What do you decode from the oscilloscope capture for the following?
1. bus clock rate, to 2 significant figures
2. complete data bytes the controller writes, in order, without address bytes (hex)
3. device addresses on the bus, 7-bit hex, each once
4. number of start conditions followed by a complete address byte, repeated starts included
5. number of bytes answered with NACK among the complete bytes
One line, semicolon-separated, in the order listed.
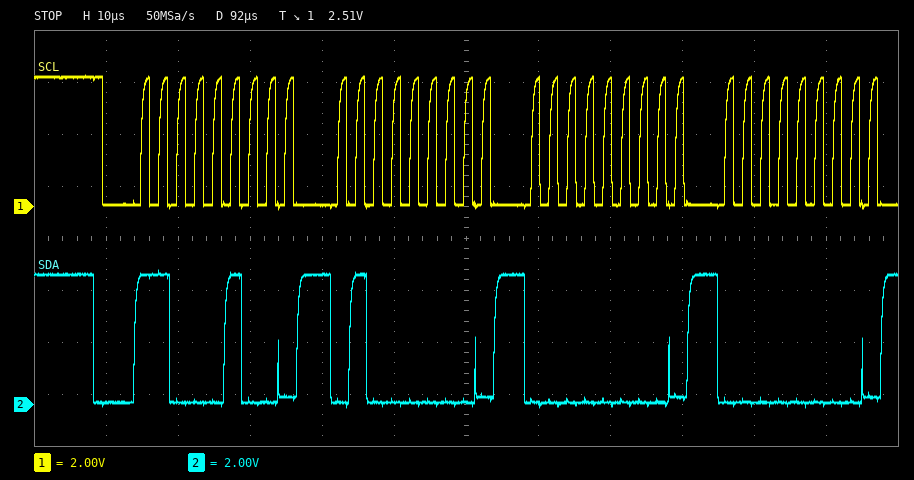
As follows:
400 kHz; 40 00 00; 0x62; 1; 0
